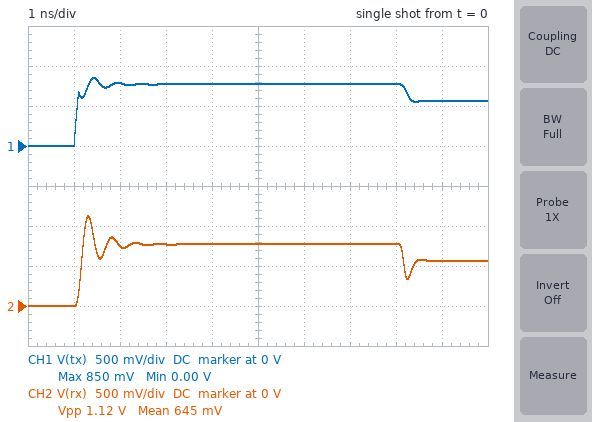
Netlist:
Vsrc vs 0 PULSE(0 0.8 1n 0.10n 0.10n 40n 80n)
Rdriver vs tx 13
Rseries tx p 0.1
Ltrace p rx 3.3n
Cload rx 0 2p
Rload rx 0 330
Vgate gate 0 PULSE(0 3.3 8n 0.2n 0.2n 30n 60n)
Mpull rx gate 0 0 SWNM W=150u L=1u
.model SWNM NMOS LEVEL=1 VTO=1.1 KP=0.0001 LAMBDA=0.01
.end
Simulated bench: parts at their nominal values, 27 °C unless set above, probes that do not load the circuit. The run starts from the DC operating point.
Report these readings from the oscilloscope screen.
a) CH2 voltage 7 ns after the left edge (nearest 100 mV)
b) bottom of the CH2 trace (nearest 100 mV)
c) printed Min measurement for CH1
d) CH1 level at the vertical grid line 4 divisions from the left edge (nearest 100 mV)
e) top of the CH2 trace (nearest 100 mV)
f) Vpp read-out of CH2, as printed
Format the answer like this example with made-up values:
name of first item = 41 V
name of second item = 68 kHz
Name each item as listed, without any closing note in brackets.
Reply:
CH2 voltage 7 ns after the left edge = 800 mV
bottom of the CH2 trace = 0 V
printed Min measurement for CH1 = 0.00 V
CH1 level at the vertical grid line 4 divisions from the left edge = 800 mV
top of the CH2 trace = 1.1 V
Vpp read-out of CH2, as printed = 1.12 V
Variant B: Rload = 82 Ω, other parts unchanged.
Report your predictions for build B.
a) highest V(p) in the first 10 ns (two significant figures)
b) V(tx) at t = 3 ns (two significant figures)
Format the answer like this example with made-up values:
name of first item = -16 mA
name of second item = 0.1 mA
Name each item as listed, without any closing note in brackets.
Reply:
highest V(p) in the first 10 ns = 720 mV
V(tx) at t = 3 ns = 690 mV
